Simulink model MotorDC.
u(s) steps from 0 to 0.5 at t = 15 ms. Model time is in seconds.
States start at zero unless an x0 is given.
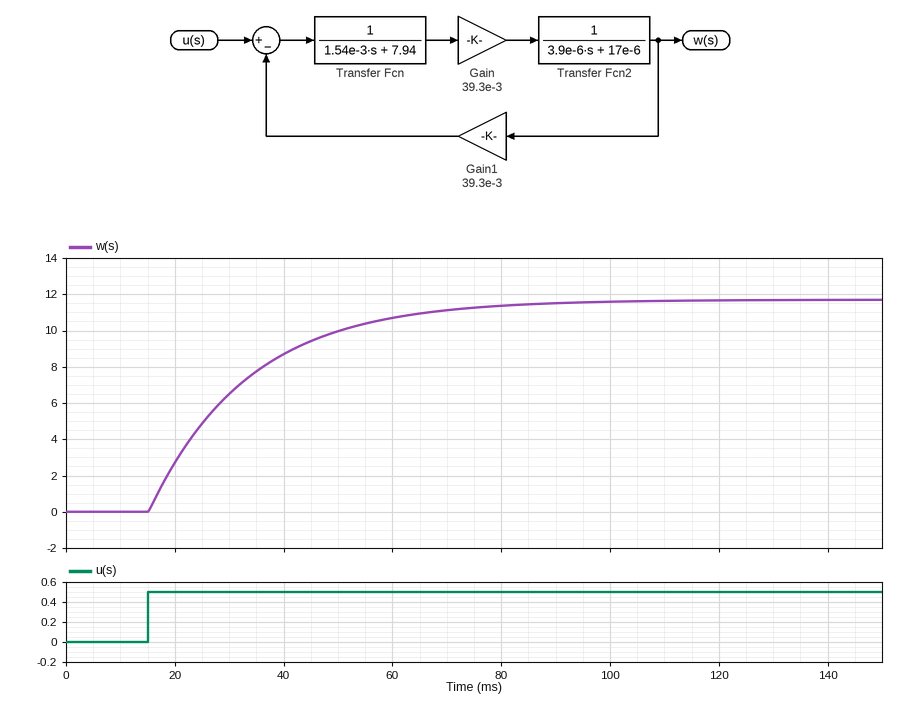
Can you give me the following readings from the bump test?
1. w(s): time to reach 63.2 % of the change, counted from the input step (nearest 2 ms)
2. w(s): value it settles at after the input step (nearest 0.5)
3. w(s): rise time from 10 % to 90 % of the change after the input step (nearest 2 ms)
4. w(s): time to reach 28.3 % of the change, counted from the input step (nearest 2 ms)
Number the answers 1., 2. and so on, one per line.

1. 18 ms
2. 11.5
3. 40 ms
4. 6 ms
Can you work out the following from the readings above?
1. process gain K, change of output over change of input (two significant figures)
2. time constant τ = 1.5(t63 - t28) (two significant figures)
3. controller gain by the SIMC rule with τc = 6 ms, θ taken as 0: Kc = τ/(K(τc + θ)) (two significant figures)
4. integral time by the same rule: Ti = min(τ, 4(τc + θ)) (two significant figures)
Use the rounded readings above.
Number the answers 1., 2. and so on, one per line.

1. 23
2. 18 ms
3. 0.13
4. 18 ms
